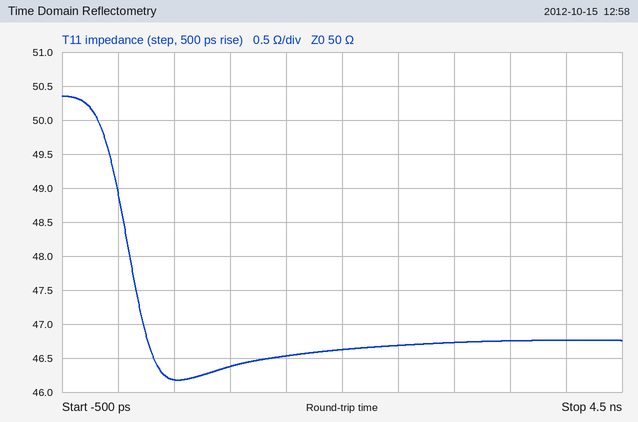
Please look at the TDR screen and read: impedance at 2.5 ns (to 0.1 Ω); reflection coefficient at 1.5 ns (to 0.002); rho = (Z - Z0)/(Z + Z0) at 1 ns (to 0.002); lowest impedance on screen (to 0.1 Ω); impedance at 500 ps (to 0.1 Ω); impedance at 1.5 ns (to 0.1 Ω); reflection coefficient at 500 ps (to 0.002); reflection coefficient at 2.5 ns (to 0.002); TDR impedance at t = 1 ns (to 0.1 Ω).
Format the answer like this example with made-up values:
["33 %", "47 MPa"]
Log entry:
["46.7 Ω", "-0.036", "-0.038", "46.2 Ω", "46.2 Ω", "46.5 Ω", "-0.040", "-0.034", "46.4 Ω"]
